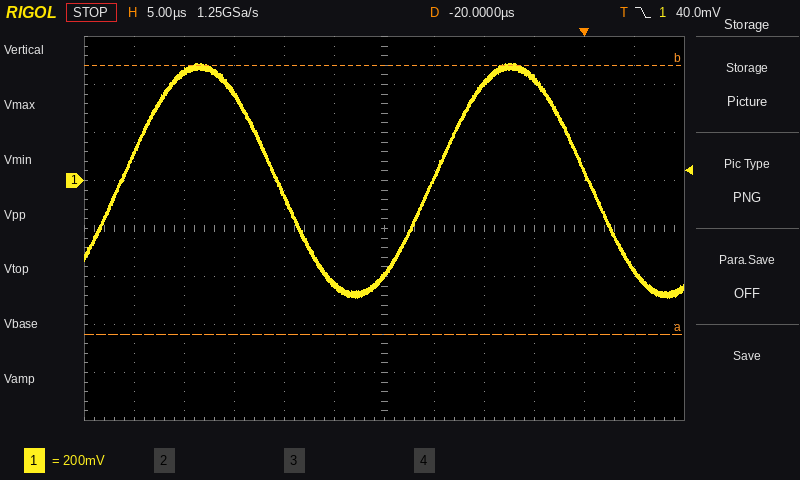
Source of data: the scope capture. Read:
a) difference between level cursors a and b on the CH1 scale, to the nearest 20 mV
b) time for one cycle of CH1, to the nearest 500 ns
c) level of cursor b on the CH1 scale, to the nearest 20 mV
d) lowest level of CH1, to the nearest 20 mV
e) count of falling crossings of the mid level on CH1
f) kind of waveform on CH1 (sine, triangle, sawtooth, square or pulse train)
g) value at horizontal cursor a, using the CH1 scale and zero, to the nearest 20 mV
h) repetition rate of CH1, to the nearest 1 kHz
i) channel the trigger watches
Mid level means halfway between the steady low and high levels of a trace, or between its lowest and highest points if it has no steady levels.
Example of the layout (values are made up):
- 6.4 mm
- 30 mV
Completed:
- 1.12 V
- 31.0 µs
- 480 mV
- -480 mV
- 2
- sine
- -640 mV
- 32 kHz
- CH1
